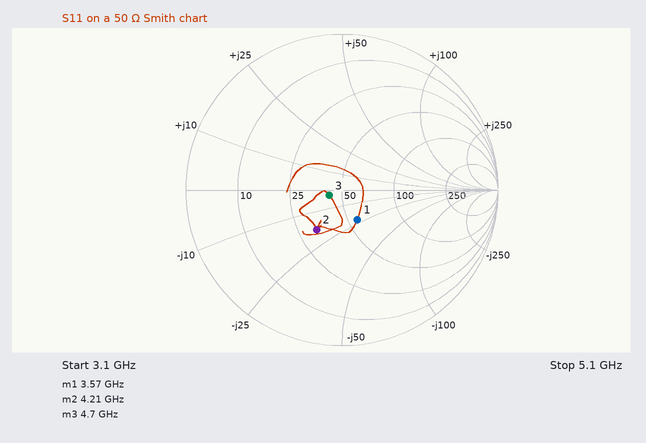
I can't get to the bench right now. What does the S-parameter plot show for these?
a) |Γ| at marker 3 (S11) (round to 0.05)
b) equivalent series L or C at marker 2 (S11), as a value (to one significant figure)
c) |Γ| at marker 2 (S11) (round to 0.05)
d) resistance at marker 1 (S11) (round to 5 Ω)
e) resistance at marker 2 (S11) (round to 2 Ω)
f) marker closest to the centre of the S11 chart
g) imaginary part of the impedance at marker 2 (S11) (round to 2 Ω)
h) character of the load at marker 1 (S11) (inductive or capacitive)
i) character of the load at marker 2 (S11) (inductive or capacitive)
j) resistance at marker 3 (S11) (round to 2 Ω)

0.10
2 pF
0.30
55 Ω
32 Ω
marker 3
-18 Ω
capacitive
capacitive
42 Ω
